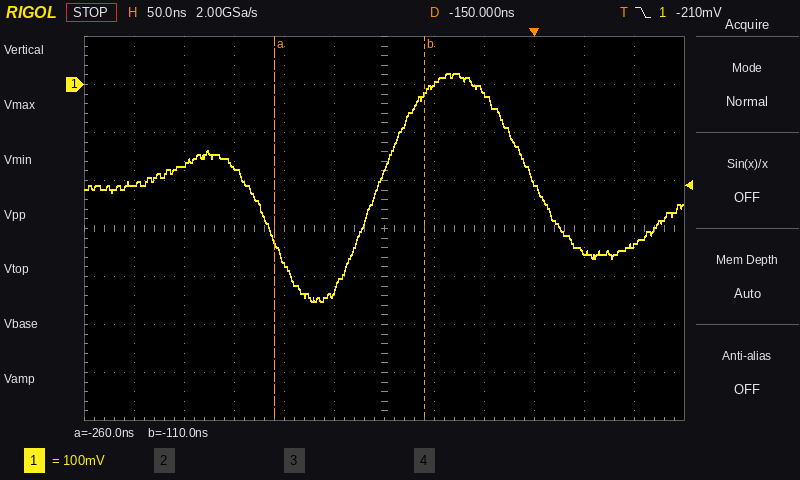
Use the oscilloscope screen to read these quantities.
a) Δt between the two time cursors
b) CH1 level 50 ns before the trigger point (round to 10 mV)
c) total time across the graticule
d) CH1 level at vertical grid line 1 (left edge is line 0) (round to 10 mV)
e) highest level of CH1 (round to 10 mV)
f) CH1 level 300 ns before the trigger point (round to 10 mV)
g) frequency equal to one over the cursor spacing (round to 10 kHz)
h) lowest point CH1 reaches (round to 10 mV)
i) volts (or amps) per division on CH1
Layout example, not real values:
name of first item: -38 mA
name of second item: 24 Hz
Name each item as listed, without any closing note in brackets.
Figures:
Δt between the two time cursors: 150 ns
CH1 level 50 ns before the trigger point: -20 mV
total time across the graticule: 600 ns
CH1 level at vertical grid line 1 (left edge is line 0): -210 mV
highest level of CH1: 20 mV
CH1 level 300 ns before the trigger point: -170 mV
frequency equal to one over the cursor spacing: 6.67 MHz
lowest point CH1 reaches: -450 mV
volts (or amps) per division on CH1: 100 mV
